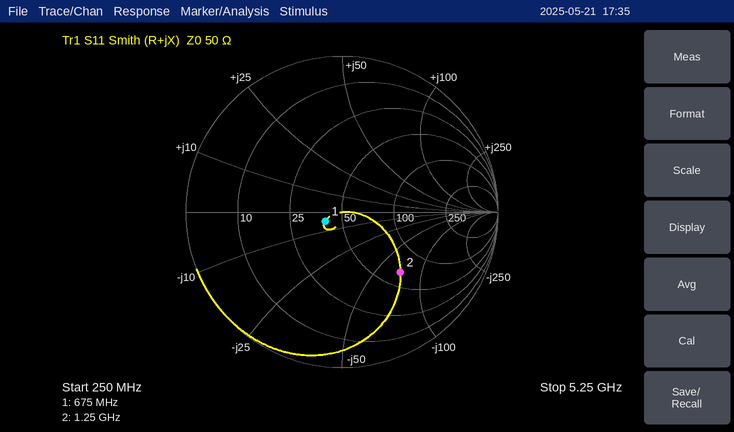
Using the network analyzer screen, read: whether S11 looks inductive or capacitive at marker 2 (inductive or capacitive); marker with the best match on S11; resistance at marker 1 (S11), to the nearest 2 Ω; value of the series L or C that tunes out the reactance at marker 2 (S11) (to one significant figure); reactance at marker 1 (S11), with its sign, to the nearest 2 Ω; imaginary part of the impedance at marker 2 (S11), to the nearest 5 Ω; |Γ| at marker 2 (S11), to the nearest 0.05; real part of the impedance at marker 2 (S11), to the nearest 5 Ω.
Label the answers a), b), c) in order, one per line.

a) capacitive
b) marker 1
c) 40 Ω
d) 9 nH
e) -4 Ω
f) -70 Ω
g) 0.55
h) 65 Ω
